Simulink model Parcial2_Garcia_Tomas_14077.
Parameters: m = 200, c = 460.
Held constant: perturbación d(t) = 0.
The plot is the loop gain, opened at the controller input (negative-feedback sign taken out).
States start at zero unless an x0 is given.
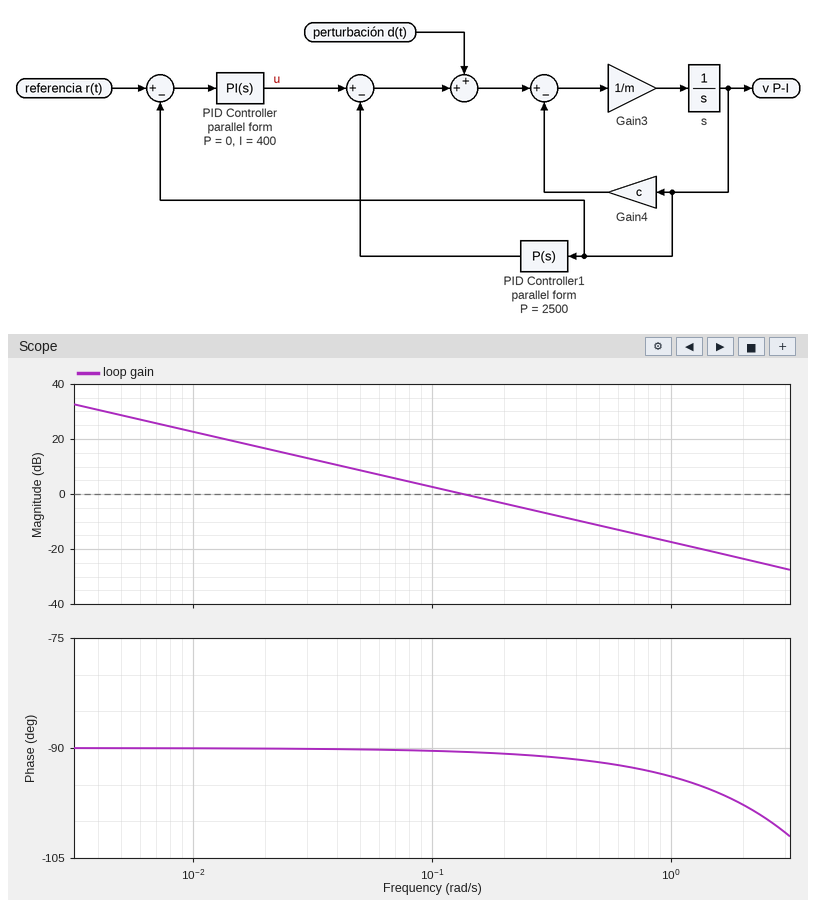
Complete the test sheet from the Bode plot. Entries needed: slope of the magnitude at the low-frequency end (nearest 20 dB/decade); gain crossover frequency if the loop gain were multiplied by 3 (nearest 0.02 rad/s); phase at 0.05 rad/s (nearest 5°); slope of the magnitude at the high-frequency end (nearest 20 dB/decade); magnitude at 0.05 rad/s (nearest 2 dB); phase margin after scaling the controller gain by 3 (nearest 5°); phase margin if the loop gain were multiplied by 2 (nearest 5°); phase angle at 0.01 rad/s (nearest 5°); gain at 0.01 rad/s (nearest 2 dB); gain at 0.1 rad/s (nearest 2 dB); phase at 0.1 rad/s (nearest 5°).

-20 dB/decade
0.40 rad/s
-90°
-20 dB/decade
8 dB
90°
90°
-90°
22 dB
2 dB
-90°
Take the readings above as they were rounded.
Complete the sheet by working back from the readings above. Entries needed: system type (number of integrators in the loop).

1
